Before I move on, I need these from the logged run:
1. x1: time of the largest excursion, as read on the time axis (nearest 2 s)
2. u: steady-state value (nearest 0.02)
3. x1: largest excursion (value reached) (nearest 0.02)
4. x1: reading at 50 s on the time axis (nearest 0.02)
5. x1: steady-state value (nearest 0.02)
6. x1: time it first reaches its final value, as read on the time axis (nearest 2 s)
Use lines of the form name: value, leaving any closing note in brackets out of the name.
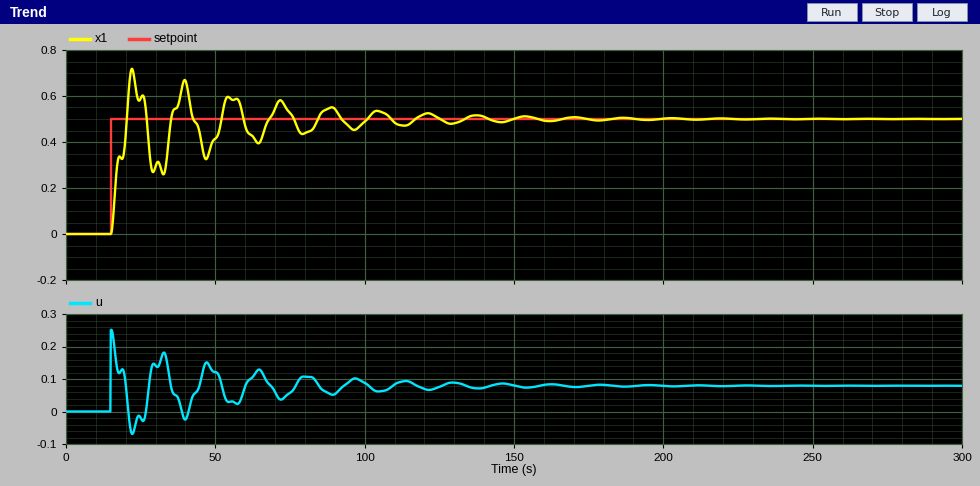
x1: time of the largest excursion, as read on the time axis: 22 s
u: steady-state value: 0.08
x1: largest excursion (value reached): 0.72
x1: reading at 50 s on the time axis: 0.42
x1: steady-state value: 0.50
x1: time it first reaches its final value, as read on the time axis: 20 s
